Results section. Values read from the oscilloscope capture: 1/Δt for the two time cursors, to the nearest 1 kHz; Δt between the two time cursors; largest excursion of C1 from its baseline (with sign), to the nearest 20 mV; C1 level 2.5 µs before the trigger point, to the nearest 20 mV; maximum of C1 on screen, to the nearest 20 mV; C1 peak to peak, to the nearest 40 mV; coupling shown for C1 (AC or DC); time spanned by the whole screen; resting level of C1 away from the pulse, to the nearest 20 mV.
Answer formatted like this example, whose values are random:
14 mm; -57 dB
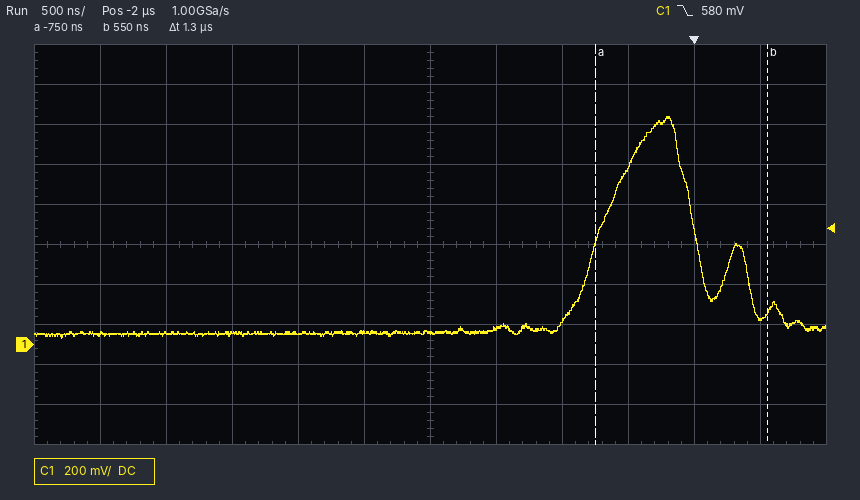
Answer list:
769 kHz; 1.3 µs; +1.08 V; 60 mV; 1.14 V; 1.12 V; DC; 6 µs; 60 mV
